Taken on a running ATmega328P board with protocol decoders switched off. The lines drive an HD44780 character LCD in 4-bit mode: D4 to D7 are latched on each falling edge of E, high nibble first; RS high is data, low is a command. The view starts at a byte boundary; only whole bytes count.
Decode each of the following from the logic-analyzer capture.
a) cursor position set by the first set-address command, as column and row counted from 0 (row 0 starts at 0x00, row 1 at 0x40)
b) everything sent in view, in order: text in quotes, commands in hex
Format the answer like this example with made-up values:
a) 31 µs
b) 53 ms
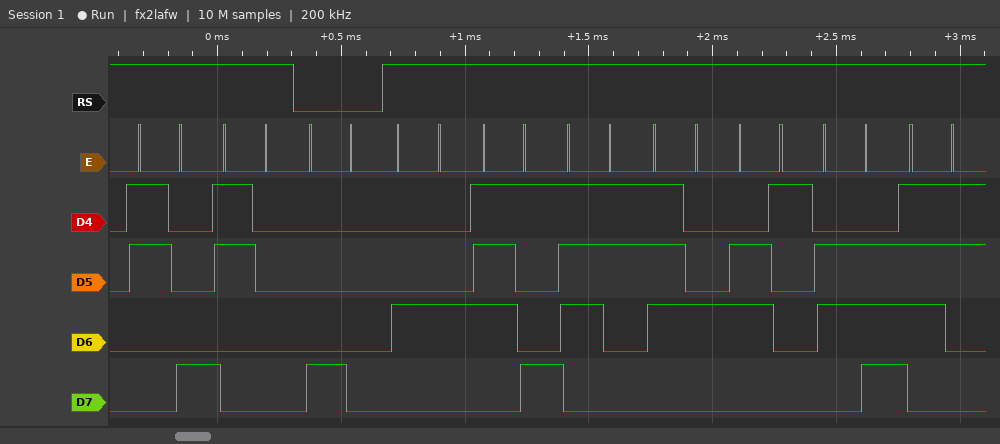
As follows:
a) column 0, row 0
b) "80" 0x80 "Dystans"
